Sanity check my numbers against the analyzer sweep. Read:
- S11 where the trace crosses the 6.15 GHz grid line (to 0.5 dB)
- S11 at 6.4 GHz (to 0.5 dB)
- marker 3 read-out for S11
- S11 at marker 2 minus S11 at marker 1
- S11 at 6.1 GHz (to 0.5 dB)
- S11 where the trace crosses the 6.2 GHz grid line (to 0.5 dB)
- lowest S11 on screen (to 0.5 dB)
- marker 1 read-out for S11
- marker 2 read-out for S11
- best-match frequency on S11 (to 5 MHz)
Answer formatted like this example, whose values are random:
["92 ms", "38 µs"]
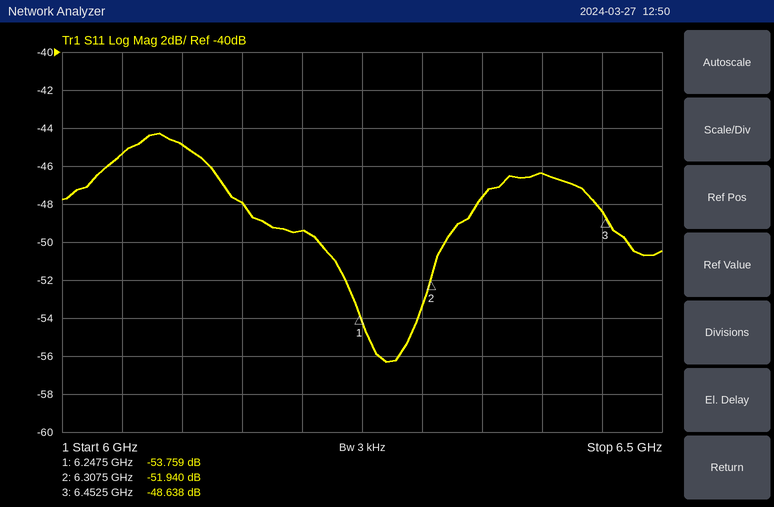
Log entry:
["-48.0 dB", "-46.5 dB", "-48.638 dB", "1.819 dB", "-45.0 dB", "-49.5 dB", "-56.5 dB", "-53.759 dB", "-51.940 dB", "6.270 GHz"]
